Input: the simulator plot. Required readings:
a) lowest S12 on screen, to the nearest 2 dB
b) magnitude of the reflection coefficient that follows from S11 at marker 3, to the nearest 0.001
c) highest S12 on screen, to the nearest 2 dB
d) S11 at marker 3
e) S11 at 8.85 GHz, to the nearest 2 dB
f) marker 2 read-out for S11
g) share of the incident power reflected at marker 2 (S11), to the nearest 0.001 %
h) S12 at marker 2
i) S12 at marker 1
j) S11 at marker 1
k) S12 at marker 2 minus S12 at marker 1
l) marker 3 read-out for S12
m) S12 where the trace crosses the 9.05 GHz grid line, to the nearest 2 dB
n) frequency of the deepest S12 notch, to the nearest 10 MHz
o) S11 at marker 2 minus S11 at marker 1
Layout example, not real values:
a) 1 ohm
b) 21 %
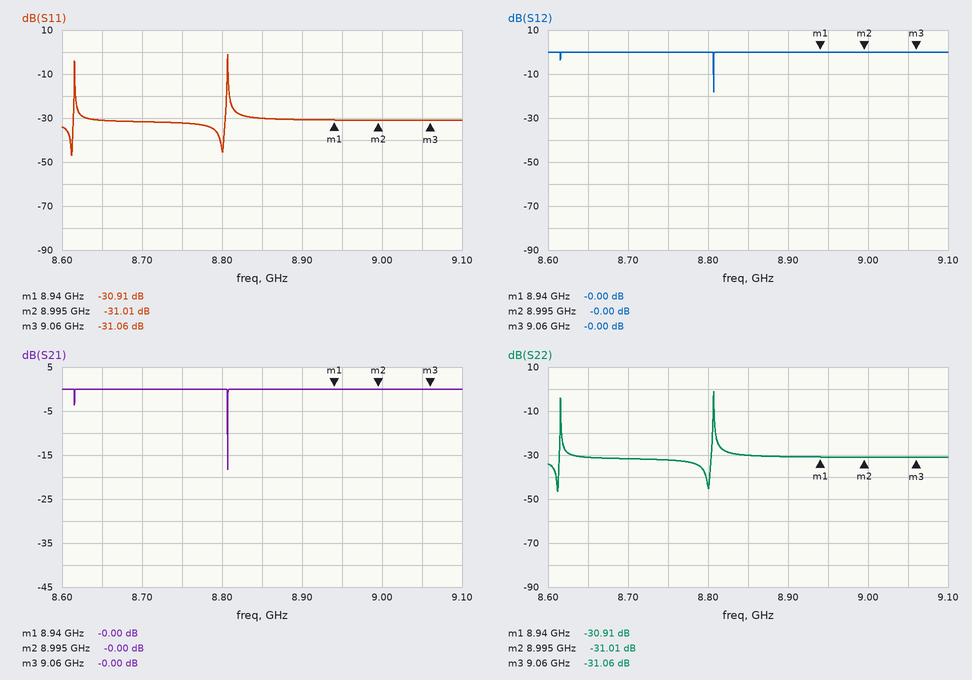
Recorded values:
a) -18 dB
b) 0.028
c) 0 dB
d) -31.06 dB
e) -30 dB
f) -31.01 dB
g) 0.079 %
h) -0.00 dB
i) -0.00 dB
j) -30.91 dB
k) 0.00 dB
l) -0.00 dB
m) 0 dB
n) 8.81 GHz
o) -0.10 dB
